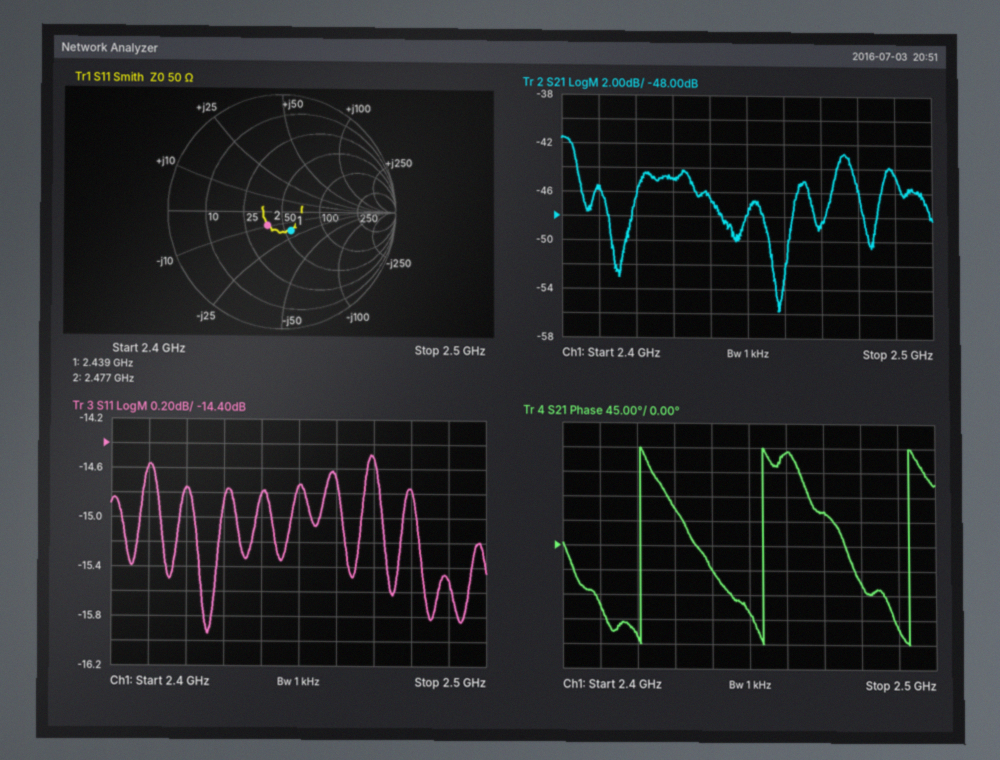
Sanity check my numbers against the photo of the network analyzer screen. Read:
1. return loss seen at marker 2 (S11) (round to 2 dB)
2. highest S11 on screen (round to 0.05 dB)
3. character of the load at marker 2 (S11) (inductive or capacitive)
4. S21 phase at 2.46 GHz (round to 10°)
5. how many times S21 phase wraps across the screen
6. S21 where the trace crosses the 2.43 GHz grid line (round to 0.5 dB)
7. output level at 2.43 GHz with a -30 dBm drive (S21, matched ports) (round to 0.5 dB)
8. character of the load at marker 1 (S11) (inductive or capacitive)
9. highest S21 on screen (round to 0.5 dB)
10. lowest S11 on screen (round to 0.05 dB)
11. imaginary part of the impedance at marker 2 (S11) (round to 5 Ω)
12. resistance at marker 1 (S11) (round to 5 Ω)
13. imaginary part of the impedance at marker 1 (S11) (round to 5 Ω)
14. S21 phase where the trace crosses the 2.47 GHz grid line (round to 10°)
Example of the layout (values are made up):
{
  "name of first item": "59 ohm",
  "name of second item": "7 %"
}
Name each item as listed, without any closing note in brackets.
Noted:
{
  "return loss seen at marker 2 (S11)": "16 dB",
  "highest S11 on screen": "-14.50 dB",
  "character of the load at marker 2 (S11)": "capacitive",
  "S21 phase at 2.46 GHz": "170°",
  "how many times S21 phase wraps across the screen": "3",
  "S21 where the trace crosses the 2.43 GHz grid line": "-45.0 dB",
  "output level at 2.43 GHz with a -30 dBm drive (S21, matched ports)": "-75.0 dBm",
  "character of the load at marker 1 (S11)": "capacitive",
  "highest S21 on screen": "-41.5 dB",
  "lowest S11 on screen": "-15.95 dB",
  "imaginary part of the impedance at marker 2 (S11)": "-10 Ω",
  "resistance at marker 1 (S11)": "55 Ω",
  "imaginary part of the impedance at marker 1 (S11)": "-20 Ω",
  "S21 phase where the trace crosses the 2.47 GHz grid line": "60°"
}
